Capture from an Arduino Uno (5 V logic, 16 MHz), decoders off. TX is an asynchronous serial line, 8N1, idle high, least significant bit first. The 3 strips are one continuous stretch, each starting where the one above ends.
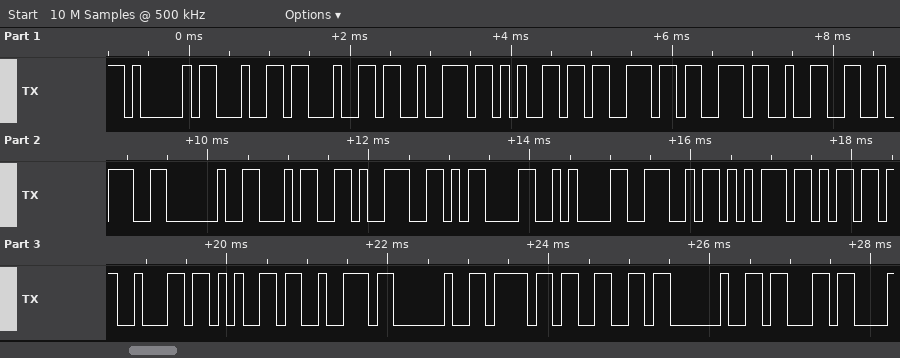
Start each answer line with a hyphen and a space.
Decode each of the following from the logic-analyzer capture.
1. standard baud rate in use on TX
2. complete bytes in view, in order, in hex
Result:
- 9600 baud
- 41 64 64 72 65 73 73 32 3A 20 34 39 0D 0A 4E 75 6D 62 65 72 20 6F 66 20 63
